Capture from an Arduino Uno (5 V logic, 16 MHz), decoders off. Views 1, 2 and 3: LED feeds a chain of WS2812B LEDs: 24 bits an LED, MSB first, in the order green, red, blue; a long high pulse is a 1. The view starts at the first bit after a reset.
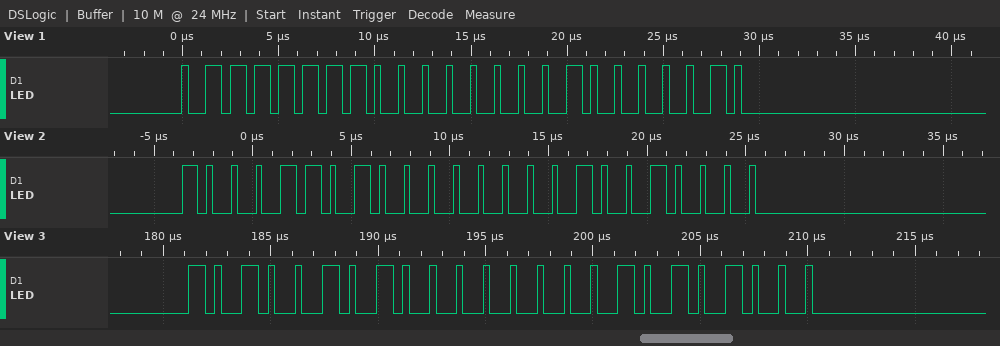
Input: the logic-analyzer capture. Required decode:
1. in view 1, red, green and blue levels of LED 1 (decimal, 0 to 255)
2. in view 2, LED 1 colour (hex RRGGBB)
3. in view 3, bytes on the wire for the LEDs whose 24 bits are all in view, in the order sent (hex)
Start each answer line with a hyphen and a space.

- 0, 127, 130
- #008D90
- A5 00 A8
